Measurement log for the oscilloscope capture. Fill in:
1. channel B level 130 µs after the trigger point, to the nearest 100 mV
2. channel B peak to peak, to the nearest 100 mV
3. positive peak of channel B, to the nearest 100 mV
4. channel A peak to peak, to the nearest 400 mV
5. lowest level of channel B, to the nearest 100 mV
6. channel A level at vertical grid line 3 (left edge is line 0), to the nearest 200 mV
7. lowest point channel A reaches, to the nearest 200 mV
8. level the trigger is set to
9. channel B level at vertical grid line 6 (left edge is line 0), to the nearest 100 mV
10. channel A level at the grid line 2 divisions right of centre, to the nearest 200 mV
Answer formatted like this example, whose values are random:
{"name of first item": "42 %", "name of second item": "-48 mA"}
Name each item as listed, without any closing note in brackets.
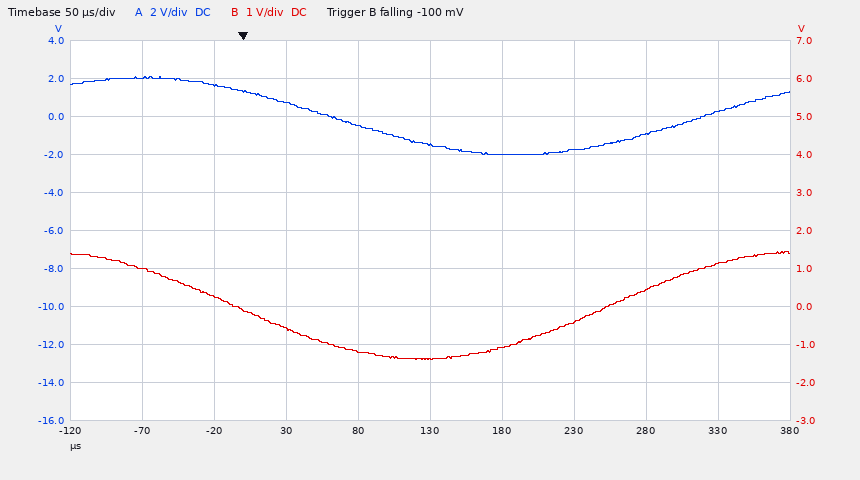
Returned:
{"channel B level 130 µs after the trigger point, to the nearest 100 mV": "-1.4 V", "channel B peak to peak, to the nearest 100 mV": "2.8 V", "positive peak of channel B, to the nearest 100 mV": "1.4 V", "channel A peak to peak, to the nearest 400 mV": "4.0 V", "lowest level of channel B, to the nearest 100 mV": "-1.4 V", "channel A level at vertical grid line 3 (left edge is line 0), to the nearest 200 mV": "800 mV", "lowest point channel A reaches, to the nearest 200 mV": "-2.0 V", "level the trigger is set to": "-100 mV", "channel B level at vertical grid line 6 (left edge is line 0), to the nearest 100 mV": "-1.1 V", "channel A level at the grid line 2 divisions right of centre, to the nearest 200 mV": "-1.8 V"}
